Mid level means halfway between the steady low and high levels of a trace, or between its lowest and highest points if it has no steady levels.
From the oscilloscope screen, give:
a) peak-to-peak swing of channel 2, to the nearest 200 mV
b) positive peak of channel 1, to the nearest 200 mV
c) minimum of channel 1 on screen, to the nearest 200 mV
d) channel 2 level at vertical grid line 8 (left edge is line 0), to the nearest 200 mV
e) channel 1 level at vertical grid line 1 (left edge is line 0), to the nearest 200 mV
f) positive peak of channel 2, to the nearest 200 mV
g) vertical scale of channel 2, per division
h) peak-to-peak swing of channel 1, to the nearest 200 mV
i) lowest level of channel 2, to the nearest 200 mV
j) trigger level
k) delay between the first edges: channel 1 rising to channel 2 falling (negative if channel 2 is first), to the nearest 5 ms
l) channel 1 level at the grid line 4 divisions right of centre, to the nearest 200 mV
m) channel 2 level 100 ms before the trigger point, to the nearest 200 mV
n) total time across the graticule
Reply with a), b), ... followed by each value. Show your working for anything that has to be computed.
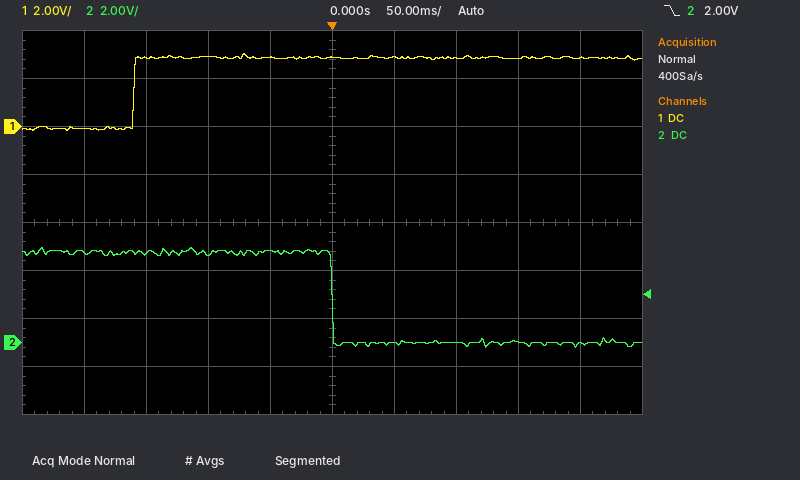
a) 4.0 V − (-200 mV) = 4.2 V
b) 3.0 V
c) -200 mV
d) 0.0 V
e) 0.0 V
f) 4.0 V
g) 2 V
h) 3.0 V − (-200 mV) = 3.2 V
i) -200 mV
j) 2.00 V
k) +160 ms
l) 2.8 V
m) 3.6 V
n) 500 ms
